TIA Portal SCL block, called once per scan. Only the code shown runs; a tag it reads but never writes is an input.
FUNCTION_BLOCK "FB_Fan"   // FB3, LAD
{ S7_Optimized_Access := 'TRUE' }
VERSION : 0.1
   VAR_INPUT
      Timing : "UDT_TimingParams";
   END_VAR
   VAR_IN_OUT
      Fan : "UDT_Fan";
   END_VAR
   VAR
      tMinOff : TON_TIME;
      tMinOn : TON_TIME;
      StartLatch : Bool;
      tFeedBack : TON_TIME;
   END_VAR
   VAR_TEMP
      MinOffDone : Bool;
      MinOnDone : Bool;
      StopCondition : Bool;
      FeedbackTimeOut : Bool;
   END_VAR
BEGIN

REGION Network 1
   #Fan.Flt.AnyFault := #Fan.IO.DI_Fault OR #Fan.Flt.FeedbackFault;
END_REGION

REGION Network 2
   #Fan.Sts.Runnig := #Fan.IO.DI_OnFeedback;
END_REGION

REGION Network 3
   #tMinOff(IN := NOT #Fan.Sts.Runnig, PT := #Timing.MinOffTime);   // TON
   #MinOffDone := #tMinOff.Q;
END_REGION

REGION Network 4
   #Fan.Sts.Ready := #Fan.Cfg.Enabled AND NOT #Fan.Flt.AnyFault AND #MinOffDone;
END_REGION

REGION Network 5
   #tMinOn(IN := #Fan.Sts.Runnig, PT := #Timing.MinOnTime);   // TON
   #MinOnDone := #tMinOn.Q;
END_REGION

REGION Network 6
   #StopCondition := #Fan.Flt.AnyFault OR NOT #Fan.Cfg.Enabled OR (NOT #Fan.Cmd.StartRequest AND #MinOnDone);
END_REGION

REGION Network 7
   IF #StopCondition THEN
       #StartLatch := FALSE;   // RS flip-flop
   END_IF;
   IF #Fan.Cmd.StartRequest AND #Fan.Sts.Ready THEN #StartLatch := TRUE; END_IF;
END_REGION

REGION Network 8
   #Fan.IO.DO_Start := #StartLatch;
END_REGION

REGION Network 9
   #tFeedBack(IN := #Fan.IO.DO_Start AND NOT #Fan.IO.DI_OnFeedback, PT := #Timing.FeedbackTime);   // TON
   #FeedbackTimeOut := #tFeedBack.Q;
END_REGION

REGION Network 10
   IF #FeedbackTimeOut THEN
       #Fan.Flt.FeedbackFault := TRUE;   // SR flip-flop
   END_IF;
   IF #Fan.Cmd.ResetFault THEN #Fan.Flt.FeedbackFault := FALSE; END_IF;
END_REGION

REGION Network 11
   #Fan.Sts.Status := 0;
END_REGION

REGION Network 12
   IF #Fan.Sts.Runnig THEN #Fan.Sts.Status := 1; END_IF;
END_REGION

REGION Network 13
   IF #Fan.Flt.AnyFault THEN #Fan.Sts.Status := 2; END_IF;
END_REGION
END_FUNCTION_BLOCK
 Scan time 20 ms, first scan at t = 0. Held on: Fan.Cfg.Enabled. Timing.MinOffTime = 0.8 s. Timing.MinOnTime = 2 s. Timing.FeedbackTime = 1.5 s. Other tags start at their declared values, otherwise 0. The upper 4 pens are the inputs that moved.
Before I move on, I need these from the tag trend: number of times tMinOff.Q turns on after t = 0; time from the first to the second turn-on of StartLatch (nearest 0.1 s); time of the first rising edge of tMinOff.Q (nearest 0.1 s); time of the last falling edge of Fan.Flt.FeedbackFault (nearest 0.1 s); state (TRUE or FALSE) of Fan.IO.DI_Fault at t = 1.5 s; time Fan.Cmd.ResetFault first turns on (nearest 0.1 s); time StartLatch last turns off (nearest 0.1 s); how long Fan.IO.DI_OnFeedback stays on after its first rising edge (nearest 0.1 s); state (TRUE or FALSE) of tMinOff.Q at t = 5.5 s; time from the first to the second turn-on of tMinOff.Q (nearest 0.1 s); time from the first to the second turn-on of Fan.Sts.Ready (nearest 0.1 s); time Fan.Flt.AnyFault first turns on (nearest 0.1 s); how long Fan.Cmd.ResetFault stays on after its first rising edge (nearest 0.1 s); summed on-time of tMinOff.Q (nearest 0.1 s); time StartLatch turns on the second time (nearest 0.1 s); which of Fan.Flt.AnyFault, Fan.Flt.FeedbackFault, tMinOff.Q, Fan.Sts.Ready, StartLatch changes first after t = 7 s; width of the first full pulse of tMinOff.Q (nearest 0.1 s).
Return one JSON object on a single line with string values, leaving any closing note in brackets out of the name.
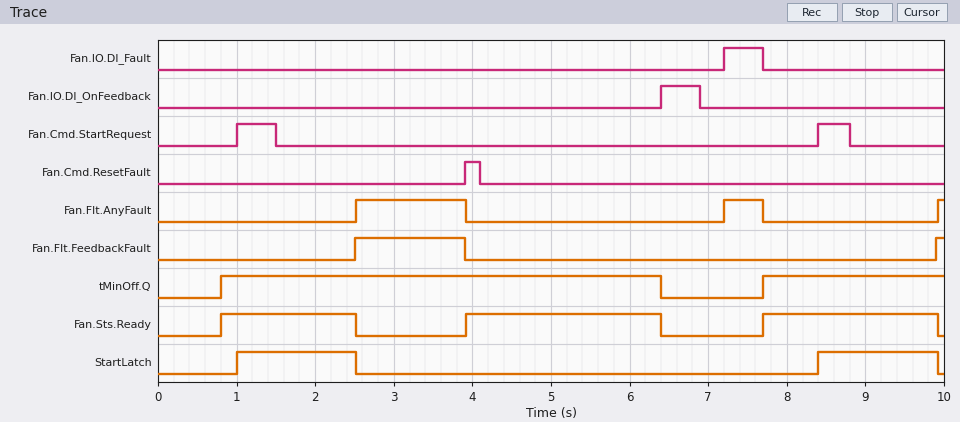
{"number of times tMinOff.Q turns on after t = 0": "2", "time from the first to the second turn-on of StartLatch": "7.4 s", "time of the first rising edge of tMinOff.Q": "0.8 s", "time of the last falling edge of Fan.Flt.FeedbackFault": "3.9 s", "state (TRUE or FALSE) of Fan.IO.DI_Fault at t = 1.5 s": "FALSE", "time Fan.Cmd.ResetFault first turns on": "3.9 s", "time StartLatch last turns off": "9.9 s", "how long Fan.IO.DI_OnFeedback stays on after its first rising edge": "0.5 s", "state (TRUE or FALSE) of tMinOff.Q at t = 5.5 s": "TRUE", "time from the first to the second turn-on of tMinOff.Q": "6.9 s", "time from the first to the second turn-on of Fan.Sts.Ready": "3.1 s", "time Fan.Flt.AnyFault first turns on": "2.5 s", "how long Fan.Cmd.ResetFault stays on after its first rising edge": "0.2 s", "summed on-time of tMinOff.Q": "7.9 s", "time StartLatch turns on the second time": "8.4 s", "which of Fan.Flt.AnyFault, Fan.Flt.FeedbackFault, tMinOff.Q, Fan.Sts.Ready, StartLatch changes first after t = 7 s": "Fan.Flt.AnyFault", "width of the first full pulse of tMinOff.Q": "5.6 s"}
